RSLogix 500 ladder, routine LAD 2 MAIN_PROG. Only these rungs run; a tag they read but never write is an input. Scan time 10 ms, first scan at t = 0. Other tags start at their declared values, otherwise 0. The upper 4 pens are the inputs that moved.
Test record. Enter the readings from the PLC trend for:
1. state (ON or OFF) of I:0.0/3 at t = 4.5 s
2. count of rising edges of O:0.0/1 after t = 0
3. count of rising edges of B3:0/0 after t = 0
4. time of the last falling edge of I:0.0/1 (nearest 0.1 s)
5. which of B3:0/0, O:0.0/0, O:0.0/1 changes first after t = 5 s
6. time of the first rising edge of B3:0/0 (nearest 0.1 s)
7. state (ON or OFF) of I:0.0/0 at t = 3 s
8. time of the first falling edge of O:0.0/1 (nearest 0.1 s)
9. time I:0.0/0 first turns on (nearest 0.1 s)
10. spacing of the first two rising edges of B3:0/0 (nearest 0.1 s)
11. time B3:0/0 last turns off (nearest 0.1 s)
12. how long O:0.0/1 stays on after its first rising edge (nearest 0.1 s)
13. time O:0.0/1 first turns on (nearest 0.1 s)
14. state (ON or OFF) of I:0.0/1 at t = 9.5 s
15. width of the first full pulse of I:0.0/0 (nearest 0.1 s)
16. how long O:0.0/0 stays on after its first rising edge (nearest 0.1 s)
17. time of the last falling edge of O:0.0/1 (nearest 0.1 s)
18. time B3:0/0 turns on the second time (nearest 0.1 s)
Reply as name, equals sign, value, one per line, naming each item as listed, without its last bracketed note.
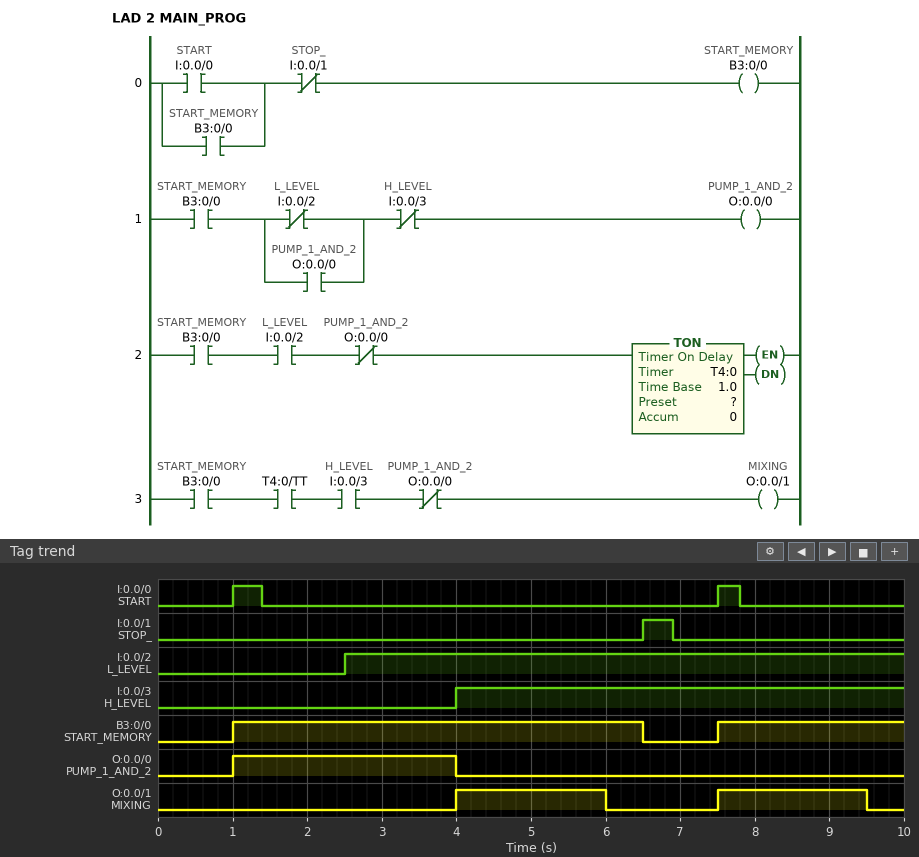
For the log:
state (ON or OFF) of I:0.0/3 at t = 4.5 s = ON
count of rising edges of O:0.0/1 after t = 0 = 2
count of rising edges of B3:0/0 after t = 0 = 2
time of the last falling edge of I:0.0/1 = 6.9 s
which of B3:0/0, O:0.0/0, O:0.0/1 changes first after t = 5 s = O:0.0/1
time of the first rising edge of B3:0/0 = 1.0 s
state (ON or OFF) of I:0.0/0 at t = 3 s = OFF
time of the first falling edge of O:0.0/1 = 6.0 s
time I:0.0/0 first turns on = 1.0 s
spacing of the first two rising edges of B3:0/0 = 6.5 s
time B3:0/0 last turns off = 6.5 s
how long O:0.0/1 stays on after its first rising edge = 2.0 s
time O:0.0/1 first turns on = 4.0 s
state (ON or OFF) of I:0.0/1 at t = 9.5 s = OFF
width of the first full pulse of I:0.0/0 = 0.4 s
how long O:0.0/0 stays on after its first rising edge = 3.0 s
time of the last falling edge of O:0.0/1 = 9.5 s
time B3:0/0 turns on the second time = 7.5 s
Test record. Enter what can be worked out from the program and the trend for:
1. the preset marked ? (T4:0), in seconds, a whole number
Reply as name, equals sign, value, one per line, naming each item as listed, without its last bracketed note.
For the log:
the preset marked ? (T4:0), in seconds, a whole number = 2 s
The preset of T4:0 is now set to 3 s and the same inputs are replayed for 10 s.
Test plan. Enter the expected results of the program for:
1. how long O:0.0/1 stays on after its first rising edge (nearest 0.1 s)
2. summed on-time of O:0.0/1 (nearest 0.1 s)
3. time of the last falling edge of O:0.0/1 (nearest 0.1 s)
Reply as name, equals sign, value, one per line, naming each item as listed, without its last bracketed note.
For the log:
how long O:0.0/1 stays on after its first rising edge = 2.5 s
summed on-time of O:0.0/1 = 5.0 s
time of the last falling edge of O:0.0/1 = 6.5 s
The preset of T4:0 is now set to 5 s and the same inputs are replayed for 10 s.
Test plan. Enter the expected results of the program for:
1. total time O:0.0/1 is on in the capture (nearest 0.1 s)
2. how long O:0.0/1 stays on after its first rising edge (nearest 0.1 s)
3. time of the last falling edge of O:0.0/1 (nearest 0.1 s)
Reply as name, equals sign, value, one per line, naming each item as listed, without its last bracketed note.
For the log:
total time O:0.0/1 is on in the capture = 5.0 s
how long O:0.0/1 stays on after its first rising edge = 2.5 s
time of the last falling edge of O:0.0/1 = 6.5 s
